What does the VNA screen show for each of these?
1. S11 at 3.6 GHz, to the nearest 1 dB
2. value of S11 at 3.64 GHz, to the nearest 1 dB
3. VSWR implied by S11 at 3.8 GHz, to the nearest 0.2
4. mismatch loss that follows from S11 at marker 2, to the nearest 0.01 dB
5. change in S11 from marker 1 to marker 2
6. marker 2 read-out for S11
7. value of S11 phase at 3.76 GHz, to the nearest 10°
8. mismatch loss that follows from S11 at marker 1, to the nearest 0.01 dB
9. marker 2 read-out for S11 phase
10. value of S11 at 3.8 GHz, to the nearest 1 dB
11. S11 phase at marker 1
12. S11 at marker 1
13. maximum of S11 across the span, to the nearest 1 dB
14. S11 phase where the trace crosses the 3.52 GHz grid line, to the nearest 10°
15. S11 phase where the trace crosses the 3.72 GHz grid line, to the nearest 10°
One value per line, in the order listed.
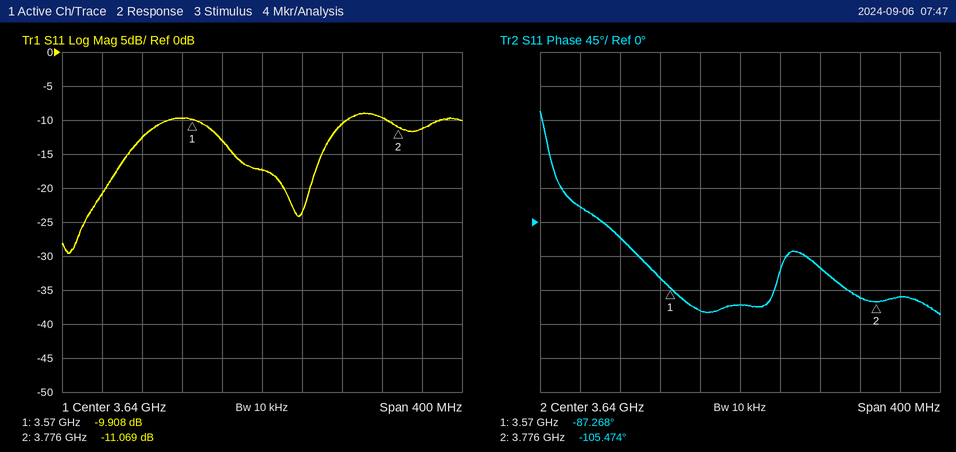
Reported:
-13 dB
-17 dB
1.8
0.35 dB
-1.161 dB
-11.069 dB
-100°
0.47 dB
-105.474°
-11 dB
-87.268°
-9.908 dB
-9 dB
-20°
-60°
